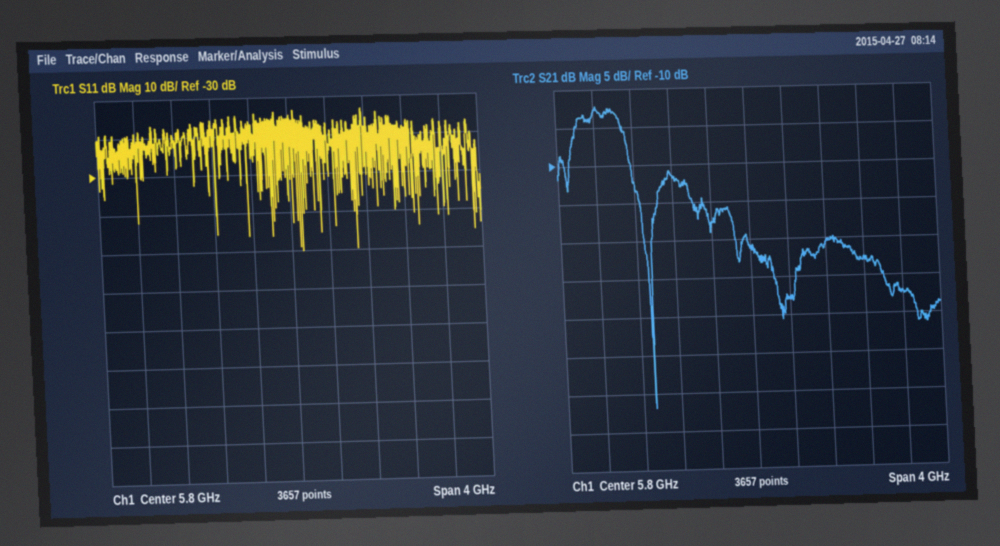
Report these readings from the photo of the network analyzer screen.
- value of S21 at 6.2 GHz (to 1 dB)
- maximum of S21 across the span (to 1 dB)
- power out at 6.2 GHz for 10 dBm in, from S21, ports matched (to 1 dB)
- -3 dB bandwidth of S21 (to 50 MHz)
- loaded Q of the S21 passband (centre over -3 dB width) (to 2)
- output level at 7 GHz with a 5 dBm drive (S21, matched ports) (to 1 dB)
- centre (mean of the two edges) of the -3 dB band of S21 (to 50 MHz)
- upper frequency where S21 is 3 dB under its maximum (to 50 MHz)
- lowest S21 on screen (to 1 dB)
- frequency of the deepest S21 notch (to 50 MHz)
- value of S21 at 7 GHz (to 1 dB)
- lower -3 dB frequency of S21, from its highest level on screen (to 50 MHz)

-28 dB
-2 dB
-18 dBm
500 MHz
8
-18 dBm
4.25 GHz
4.50 GHz
-42 dB
4.75 GHz
-23 dB
4.00 GHz
